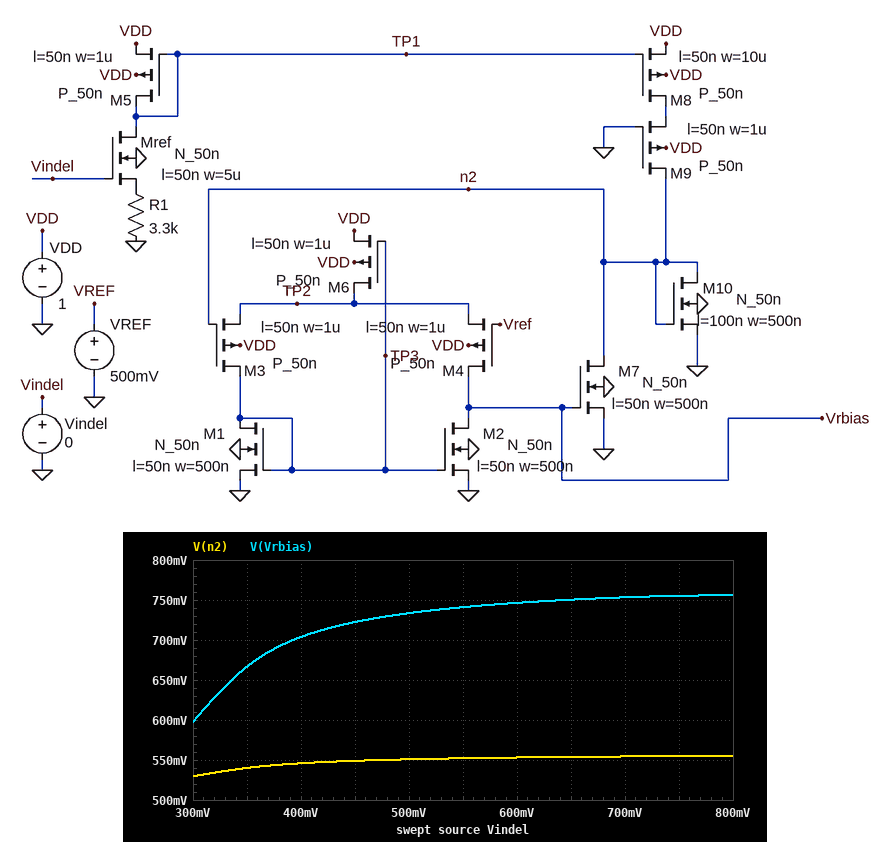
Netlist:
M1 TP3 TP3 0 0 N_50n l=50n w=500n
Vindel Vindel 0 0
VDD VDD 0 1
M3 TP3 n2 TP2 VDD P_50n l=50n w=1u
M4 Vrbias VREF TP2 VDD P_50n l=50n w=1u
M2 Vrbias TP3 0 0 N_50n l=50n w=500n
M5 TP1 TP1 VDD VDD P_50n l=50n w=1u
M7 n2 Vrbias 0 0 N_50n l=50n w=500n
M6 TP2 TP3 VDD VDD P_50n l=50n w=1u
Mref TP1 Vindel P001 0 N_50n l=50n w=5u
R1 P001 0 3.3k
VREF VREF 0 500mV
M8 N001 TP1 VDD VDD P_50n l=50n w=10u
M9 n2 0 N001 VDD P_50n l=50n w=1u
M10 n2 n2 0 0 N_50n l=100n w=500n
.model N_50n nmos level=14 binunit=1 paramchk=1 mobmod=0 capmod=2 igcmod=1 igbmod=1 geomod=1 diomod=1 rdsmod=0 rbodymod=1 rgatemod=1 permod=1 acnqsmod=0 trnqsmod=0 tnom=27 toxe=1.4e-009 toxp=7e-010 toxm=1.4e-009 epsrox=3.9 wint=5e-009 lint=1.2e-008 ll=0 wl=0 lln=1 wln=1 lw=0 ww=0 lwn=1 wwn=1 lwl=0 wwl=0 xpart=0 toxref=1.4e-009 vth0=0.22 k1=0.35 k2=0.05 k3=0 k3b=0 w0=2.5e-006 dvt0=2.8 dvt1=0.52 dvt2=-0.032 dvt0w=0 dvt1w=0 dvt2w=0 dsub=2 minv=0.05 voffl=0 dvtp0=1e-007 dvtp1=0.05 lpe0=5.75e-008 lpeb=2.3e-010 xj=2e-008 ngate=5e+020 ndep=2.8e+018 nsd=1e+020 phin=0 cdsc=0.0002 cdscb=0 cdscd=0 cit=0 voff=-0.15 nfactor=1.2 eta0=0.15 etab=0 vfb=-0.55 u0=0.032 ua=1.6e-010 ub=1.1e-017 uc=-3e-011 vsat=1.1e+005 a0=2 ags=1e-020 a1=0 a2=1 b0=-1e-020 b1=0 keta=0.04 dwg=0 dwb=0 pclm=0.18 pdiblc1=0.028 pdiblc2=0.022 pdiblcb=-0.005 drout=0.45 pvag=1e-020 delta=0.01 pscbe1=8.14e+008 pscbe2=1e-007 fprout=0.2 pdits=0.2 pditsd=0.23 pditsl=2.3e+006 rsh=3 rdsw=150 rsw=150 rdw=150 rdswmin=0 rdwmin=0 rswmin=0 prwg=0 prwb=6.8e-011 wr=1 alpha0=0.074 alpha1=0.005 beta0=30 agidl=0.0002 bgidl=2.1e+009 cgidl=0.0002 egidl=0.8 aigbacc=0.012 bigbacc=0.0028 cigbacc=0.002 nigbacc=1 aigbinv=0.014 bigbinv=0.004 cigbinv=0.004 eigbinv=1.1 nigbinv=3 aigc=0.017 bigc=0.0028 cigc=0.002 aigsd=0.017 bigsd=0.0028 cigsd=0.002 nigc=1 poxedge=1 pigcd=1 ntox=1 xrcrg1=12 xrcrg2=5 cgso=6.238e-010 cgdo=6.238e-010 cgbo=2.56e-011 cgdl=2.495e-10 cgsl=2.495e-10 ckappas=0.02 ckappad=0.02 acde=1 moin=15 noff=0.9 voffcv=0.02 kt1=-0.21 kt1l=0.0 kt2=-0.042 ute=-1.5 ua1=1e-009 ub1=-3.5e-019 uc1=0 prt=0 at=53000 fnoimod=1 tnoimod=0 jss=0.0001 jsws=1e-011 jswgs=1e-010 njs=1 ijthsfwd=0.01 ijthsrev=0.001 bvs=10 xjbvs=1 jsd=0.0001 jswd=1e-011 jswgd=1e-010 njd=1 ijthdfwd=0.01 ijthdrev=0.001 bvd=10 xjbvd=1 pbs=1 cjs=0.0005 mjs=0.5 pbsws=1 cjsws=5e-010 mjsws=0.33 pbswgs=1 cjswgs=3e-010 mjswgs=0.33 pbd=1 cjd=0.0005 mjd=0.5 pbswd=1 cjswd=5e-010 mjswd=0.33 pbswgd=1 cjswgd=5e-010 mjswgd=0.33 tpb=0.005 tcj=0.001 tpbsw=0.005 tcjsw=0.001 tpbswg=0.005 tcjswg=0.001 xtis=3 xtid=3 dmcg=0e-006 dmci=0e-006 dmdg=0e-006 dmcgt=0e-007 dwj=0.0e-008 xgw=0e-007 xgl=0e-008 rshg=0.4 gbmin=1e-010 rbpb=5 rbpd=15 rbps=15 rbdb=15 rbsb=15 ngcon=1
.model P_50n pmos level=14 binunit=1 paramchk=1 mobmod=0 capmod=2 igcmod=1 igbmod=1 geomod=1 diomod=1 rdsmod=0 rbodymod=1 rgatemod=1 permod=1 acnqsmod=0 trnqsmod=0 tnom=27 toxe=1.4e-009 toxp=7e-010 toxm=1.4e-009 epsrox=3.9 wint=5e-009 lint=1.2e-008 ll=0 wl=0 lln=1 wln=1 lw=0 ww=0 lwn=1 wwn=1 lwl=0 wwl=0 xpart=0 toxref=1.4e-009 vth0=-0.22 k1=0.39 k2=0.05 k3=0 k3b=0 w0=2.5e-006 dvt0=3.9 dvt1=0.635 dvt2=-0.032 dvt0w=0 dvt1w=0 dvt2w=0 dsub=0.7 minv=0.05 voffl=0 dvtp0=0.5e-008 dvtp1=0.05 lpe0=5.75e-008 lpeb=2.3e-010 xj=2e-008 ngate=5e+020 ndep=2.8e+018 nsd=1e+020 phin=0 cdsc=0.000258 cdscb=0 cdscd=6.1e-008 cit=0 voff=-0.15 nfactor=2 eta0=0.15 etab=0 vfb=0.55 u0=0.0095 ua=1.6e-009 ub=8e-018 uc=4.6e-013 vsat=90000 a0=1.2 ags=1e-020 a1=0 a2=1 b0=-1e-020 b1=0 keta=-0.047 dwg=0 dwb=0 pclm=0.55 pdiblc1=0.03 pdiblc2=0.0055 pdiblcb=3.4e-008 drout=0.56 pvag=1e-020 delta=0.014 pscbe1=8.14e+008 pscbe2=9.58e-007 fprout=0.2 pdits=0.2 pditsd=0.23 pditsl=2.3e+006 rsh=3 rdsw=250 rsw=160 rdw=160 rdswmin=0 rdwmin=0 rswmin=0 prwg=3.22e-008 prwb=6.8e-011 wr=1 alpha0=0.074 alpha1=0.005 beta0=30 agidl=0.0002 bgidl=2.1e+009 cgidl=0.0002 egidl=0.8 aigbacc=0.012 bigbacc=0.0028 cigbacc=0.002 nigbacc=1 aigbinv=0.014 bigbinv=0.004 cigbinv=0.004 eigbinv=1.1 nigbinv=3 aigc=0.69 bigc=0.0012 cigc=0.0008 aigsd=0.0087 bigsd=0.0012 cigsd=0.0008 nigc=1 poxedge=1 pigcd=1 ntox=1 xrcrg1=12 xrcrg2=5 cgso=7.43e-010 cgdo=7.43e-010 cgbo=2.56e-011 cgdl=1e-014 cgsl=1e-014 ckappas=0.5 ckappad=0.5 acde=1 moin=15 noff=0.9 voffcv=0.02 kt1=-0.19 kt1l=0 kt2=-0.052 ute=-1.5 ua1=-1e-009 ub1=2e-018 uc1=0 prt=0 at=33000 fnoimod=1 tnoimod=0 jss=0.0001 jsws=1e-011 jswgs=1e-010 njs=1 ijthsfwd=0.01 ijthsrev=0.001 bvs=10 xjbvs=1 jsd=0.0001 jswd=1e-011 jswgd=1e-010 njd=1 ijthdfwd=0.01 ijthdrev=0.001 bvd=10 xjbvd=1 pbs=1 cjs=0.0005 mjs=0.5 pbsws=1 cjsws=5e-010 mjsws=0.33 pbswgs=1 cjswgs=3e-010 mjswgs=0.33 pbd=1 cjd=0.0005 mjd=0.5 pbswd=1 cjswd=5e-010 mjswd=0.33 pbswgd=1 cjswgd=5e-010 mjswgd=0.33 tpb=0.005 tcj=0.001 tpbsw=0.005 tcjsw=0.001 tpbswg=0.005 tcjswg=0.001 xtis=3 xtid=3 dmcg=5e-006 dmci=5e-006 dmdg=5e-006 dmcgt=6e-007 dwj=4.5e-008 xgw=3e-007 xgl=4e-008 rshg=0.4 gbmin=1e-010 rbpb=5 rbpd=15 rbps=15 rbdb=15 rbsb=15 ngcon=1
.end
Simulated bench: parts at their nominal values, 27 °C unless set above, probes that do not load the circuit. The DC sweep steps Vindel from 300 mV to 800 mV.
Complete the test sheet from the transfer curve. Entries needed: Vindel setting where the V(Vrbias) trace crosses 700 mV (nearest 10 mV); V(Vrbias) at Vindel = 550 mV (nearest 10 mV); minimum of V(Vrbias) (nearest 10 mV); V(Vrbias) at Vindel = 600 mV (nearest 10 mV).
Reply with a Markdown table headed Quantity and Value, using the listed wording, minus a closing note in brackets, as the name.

| Quantity | Value |
|---|---|
| Vindel setting where the V(Vrbias) trace crosses 700 mV | 390 mV |
| V(Vrbias) at Vindel = 550 mV | 740 mV |
| minimum of V(Vrbias) | 600 mV |
| V(Vrbias) at Vindel = 600 mV | 750 mV |
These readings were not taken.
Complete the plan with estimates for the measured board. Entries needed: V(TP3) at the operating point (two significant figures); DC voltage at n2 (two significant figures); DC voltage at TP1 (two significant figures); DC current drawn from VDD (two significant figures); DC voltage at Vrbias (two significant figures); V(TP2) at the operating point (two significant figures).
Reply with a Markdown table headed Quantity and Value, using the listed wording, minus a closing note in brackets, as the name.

| Quantity | Value |
|---|---|
| V(TP3) at the operating point | 460 mV |
| DC voltage at n2 | 320 mV |
| DC voltage at TP1 | 870 mV |
| DC current drawn from VDD | 43 µA |
| DC voltage at Vrbias | 16 mV |
| V(TP2) at the operating point | 830 mV |
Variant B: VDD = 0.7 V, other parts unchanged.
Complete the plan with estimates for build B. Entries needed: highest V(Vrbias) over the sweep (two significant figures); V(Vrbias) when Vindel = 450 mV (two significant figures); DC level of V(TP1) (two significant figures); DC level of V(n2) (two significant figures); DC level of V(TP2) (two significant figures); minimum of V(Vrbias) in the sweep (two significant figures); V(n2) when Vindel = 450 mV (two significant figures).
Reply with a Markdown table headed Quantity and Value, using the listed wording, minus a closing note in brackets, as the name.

| Quantity | Value |
|---|---|
| highest V(Vrbias) over the sweep | 470 mV |
| V(Vrbias) when Vindel = 450 mV | 460 mV |
| DC level of V(TP1) | 590 mV |
| DC level of V(n2) | 280 mV |
| DC level of V(TP2) | 630 mV |
| minimum of V(Vrbias) in the sweep | 440 mV |
| V(n2) when Vindel = 450 mV | 540 mV |
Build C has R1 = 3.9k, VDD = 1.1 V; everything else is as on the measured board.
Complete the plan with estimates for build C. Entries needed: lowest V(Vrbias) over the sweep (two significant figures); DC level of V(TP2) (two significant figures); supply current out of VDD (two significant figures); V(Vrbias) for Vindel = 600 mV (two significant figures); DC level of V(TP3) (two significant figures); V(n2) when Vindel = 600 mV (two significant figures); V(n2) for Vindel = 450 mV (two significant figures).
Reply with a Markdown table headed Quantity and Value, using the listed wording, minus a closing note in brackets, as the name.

| Quantity | Value |
|---|---|
| lowest V(Vrbias) over the sweep | 610 mV |
| DC level of V(TP2) | 890 mV |
| supply current out of VDD | 66 µA |
| V(Vrbias) for Vindel = 600 mV | 820 mV |
| DC level of V(TP3) | 490 mV |
| V(n2) when Vindel = 600 mV | 570 mV |
| V(n2) for Vindel = 450 mV | 560 mV |
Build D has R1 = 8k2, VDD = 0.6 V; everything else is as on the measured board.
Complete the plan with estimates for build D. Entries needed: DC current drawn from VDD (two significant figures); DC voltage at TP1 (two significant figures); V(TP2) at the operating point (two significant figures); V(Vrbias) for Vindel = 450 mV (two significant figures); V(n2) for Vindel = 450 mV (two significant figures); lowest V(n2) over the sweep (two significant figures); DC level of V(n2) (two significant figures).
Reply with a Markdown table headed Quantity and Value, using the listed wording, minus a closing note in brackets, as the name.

| Quantity | Value |
|---|---|
| DC current drawn from VDD | 2.3 µA |
| DC voltage at TP1 | 500 mV |
| V(TP2) at the operating point | 560 mV |
| V(Vrbias) for Vindel = 450 mV | 290 mV |
| V(n2) for Vindel = 450 mV | 530 mV |
| lowest V(n2) over the sweep | 520 mV |
| DC level of V(n2) | 270 mV |
